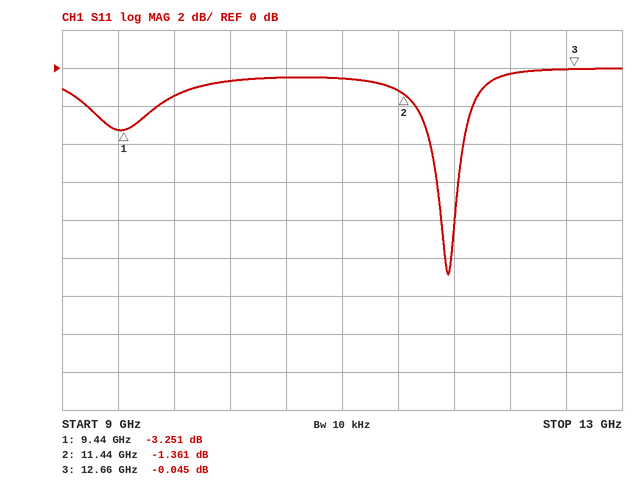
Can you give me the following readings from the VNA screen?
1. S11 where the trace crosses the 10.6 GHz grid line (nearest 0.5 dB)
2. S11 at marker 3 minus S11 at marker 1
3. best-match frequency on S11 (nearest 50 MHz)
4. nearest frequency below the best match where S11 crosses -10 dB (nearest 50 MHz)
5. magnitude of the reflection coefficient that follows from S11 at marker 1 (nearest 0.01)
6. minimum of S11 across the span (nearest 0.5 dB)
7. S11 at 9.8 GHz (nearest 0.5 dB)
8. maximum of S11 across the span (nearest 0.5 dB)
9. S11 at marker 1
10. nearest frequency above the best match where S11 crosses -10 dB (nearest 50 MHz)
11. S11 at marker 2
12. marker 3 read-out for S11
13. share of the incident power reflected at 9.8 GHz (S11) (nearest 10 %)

-0.5 dB
3.206 dB
11.75 GHz
11.75 GHz
0.69
-11.0 dB
-1.5 dB
0.0 dB
-3.251 dB
11.80 GHz
-1.361 dB
-0.045 dB
70 %
